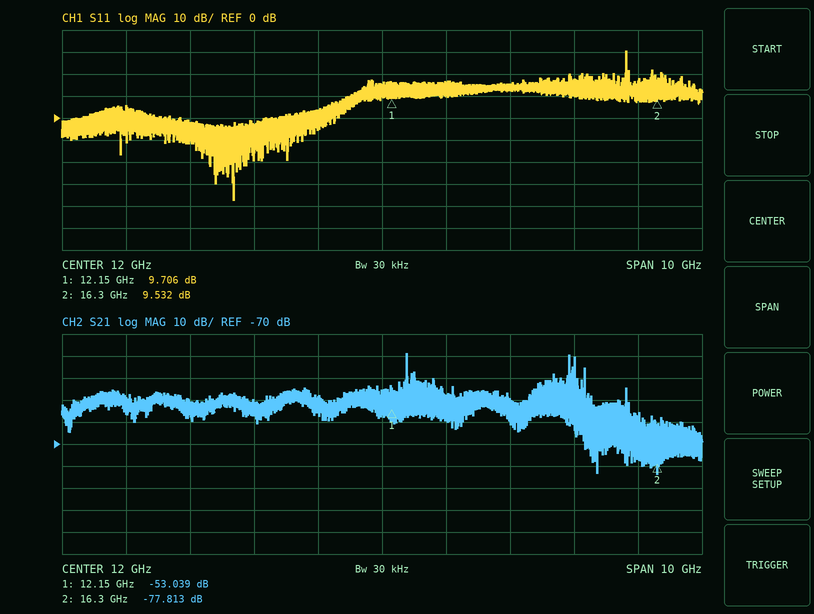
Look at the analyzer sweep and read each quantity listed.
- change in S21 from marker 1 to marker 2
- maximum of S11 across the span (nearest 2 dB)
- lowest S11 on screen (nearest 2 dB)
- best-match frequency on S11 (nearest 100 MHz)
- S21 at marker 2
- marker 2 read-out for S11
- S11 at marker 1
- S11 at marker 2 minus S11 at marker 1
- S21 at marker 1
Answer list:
-24.774 dB
30 dB
-38 dB
9.7 GHz
-77.813 dB
9.532 dB
9.706 dB
-0.174 dB
-53.039 dB
